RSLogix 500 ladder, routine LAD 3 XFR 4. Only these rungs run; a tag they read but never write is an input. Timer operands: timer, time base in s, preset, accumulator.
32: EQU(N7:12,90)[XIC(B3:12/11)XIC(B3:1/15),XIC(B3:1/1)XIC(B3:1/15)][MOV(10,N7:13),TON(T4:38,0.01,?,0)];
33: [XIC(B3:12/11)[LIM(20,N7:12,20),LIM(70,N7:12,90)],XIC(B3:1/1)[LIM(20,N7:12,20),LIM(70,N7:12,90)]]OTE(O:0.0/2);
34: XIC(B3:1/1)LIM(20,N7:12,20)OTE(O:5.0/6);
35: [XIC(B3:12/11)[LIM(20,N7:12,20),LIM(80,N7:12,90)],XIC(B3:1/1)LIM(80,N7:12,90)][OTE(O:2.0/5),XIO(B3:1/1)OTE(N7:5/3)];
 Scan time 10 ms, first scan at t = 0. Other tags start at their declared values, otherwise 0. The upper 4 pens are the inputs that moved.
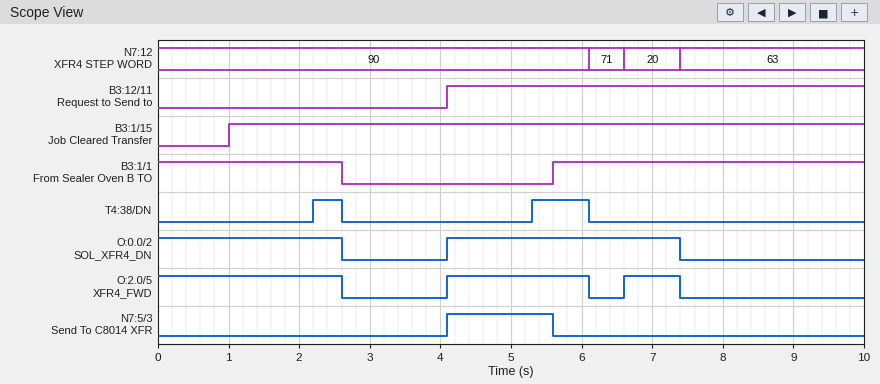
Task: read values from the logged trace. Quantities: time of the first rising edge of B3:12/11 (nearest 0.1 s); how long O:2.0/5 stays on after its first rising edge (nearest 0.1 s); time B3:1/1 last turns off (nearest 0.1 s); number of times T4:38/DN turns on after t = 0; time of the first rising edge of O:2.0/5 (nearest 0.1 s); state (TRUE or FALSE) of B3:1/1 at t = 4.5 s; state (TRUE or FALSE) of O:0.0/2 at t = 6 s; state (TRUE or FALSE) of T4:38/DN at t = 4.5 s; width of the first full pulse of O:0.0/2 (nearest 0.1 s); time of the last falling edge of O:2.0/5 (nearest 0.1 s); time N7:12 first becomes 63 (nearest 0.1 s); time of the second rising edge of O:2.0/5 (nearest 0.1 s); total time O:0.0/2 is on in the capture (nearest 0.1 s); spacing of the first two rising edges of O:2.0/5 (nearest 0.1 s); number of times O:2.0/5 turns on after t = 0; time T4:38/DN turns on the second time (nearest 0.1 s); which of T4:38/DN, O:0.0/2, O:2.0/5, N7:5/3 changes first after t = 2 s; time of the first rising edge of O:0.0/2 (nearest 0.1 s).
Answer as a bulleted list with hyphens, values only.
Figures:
- 4.1 s
- 2.0 s
- 2.6 s
- 2
- 4.1 s
- FALSE
- TRUE
- FALSE
- 3.3 s
- 7.4 s
- 7.4 s
- 6.6 s
- 5.9 s
- 2.5 s
- 2
- 5.3 s
- T4:38/DN
- 4.1 s
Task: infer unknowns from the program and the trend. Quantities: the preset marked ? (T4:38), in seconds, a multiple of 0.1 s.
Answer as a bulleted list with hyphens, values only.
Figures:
- 1.2 s
